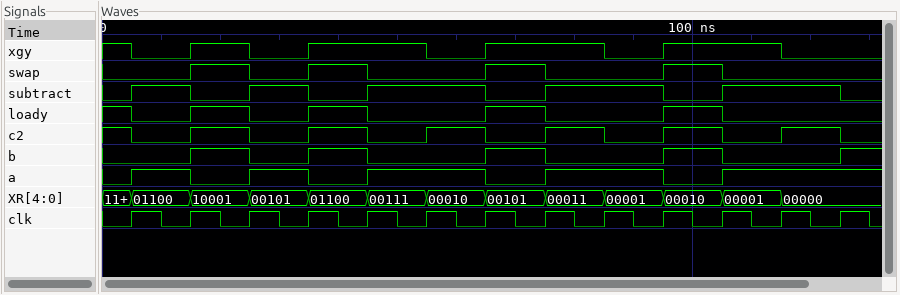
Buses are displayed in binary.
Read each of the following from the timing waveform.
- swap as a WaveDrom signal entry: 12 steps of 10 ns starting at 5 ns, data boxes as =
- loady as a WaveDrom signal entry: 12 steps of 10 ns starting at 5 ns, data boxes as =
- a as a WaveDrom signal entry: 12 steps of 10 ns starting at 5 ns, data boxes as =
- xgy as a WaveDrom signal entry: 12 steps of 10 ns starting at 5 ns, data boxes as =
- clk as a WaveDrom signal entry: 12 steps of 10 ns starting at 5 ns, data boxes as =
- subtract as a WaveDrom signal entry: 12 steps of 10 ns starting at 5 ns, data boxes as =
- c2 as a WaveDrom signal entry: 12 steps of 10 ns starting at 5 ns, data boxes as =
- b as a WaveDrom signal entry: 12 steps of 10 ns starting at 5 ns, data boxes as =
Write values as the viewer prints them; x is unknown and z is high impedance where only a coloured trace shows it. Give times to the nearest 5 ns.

{name: 'swap', wave: '01010.10.10.'}
{name: 'loady', wave: '01010.10.10.'}
{name: 'a', wave: '10101.01.01.'}
{name: 'xgy', wave: '0101.01.01.0'}
{name: 'clk', wave: 'p...........'}
{name: 'subtract', wave: '10101.01.01.'}
{name: 'c2', wave: '010101010101'}
{name: 'b', wave: '01010.10.10.'}
